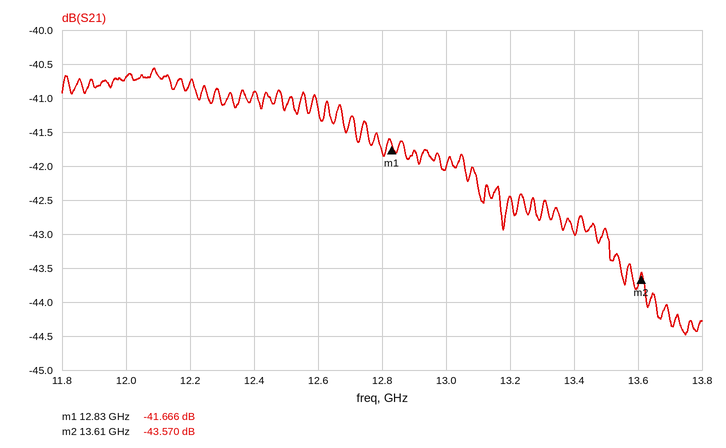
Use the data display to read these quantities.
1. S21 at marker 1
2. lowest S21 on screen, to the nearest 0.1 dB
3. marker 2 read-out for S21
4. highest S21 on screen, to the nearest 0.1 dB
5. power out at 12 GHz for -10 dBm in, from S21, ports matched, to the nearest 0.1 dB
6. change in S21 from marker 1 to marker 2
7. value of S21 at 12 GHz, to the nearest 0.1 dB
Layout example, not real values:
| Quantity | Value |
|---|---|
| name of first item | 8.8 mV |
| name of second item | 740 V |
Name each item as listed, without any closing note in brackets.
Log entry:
| Quantity | Value |
|---|---|
| S21 at marker 1 | -41.666 dB |
| lowest S21 on screen, to the nearest 0.1 dB | -44.5 dB |
| marker 2 read-out for S21 | -43.570 dB |
| highest S21 on screen, to the nearest 0.1 dB | -40.6 dB |
| power out at 12 GHz for -10 dBm in, from S21, ports matched, to the nearest 0.1 dB | -50.7 dBm |
| change in S21 from marker 1 to marker 2 | -1.904 dB |
| value of S21 at 12 GHz, to the nearest 0.1 dB | -40.7 dB |
